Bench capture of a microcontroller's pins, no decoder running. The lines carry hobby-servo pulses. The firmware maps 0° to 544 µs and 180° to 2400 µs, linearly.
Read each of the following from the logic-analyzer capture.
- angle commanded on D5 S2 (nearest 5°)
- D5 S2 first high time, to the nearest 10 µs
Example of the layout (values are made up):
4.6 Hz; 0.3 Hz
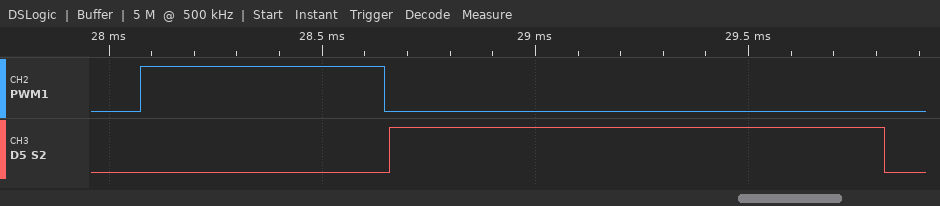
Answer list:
60°; 1160 µs
